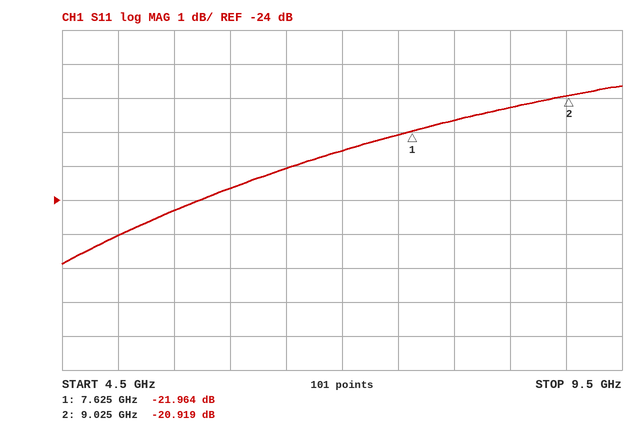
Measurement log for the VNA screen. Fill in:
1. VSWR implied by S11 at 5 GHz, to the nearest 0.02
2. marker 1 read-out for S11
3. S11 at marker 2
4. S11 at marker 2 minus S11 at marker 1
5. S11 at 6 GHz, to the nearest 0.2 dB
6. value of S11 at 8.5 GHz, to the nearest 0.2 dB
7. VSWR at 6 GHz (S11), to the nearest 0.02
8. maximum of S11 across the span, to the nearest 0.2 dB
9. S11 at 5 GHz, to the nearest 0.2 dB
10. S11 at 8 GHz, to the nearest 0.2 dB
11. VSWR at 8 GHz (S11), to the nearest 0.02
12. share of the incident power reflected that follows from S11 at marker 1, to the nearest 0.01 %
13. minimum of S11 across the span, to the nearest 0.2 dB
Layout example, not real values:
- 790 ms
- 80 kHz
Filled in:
- 1.12
- -21.964 dB
- -20.919 dB
- 1.045 dB
- -23.6 dB
- -21.2 dB
- 1.14
- -20.6 dB
- -25.0 dB
- -21.6 dB
- 1.18
- 0.64 %
- -25.8 dB
